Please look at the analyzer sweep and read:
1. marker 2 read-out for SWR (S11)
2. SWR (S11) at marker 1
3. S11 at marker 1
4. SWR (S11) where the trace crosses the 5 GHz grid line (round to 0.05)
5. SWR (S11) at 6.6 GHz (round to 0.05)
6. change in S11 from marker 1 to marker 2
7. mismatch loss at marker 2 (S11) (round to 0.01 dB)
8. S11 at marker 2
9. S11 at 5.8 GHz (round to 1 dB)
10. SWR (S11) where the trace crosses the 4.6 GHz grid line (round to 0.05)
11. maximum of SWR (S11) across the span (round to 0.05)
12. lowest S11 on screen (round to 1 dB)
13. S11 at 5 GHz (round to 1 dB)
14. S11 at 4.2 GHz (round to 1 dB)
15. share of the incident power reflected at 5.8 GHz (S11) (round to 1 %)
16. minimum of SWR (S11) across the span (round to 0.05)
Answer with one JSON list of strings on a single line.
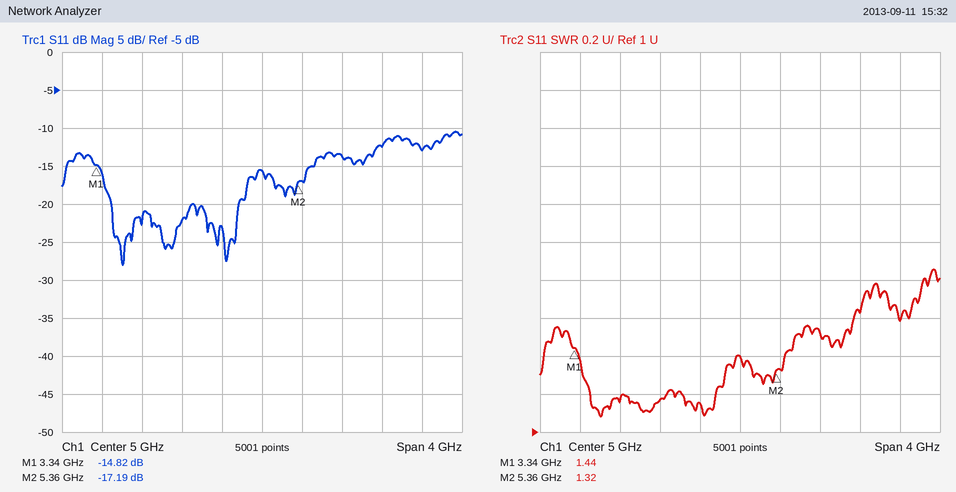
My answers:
["1.32", "1.44", "-14.82 dB", "1.40", "1.60", "-2.37 dB", "0.08 dB", "-17.19 dB", "-14 dB", "1.15", "1.85", "-28 dB", "-16 dB", "-22 dB", "4 %", "1.10"]
